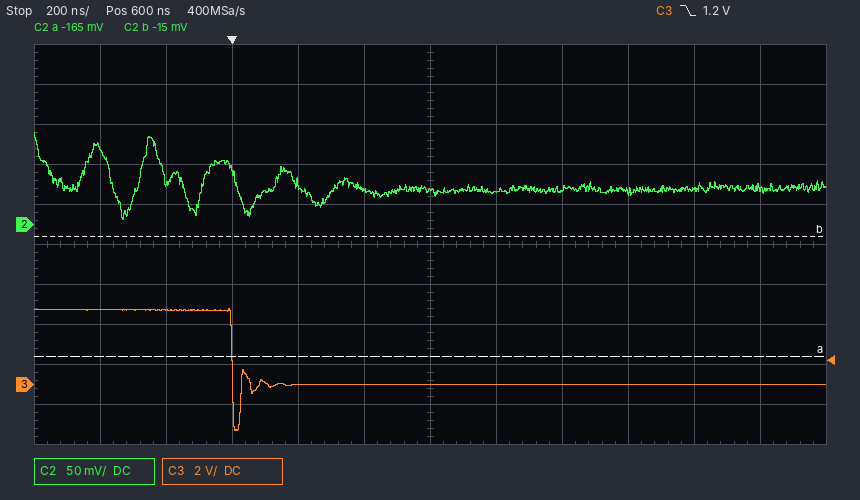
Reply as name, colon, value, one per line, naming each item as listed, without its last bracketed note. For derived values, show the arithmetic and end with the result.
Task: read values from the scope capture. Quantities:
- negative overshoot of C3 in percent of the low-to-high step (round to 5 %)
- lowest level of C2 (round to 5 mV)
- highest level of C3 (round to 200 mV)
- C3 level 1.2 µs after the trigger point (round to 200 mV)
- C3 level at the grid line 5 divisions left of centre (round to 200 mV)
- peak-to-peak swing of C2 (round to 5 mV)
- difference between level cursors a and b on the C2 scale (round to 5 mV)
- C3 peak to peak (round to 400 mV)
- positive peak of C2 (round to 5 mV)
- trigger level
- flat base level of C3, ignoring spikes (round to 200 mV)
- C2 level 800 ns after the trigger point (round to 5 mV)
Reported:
negative overshoot of C3 in percent of the low-to-high step: 60 %
lowest level of C2: 5 mV
highest level of C3: 3.8 V
C3 level 1.2 µs after the trigger point: 0.0 V
C3 level at the grid line 5 divisions left of centre: 3.8 V
peak-to-peak swing of C2: 115 mV − (5 mV) = 110 mV
difference between level cursors a and b on the C2 scale: 150 mV
C3 peak to peak: 6.0 V
positive peak of C2: 115 mV
trigger level: 1.2 V
flat base level of C3, ignoring spikes: 0.0 V
C2 level 800 ns after the trigger point: 40 mV
